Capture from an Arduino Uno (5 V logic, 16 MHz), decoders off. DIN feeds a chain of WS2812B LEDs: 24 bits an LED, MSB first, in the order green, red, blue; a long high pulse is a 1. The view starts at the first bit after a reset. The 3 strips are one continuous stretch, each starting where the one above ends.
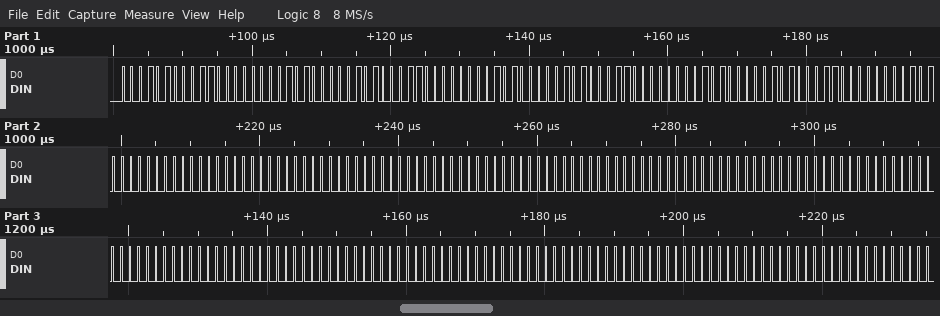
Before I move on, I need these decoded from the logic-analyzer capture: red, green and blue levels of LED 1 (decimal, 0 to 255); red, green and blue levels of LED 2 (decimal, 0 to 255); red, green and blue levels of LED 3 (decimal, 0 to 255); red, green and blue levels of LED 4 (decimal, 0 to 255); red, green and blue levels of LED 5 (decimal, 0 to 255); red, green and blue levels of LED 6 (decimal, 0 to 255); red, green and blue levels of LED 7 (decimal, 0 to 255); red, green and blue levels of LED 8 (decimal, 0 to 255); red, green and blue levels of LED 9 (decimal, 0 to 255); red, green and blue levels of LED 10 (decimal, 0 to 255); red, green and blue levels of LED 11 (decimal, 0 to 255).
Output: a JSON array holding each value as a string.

["96, 20, 20", "96, 20, 20", "96, 20, 20", "96, 20, 20", "0, 0, 0", "0, 0, 0", "0, 0, 0", "0, 0, 0", "0, 0, 0", "0, 0, 0", "0, 0, 0"]
